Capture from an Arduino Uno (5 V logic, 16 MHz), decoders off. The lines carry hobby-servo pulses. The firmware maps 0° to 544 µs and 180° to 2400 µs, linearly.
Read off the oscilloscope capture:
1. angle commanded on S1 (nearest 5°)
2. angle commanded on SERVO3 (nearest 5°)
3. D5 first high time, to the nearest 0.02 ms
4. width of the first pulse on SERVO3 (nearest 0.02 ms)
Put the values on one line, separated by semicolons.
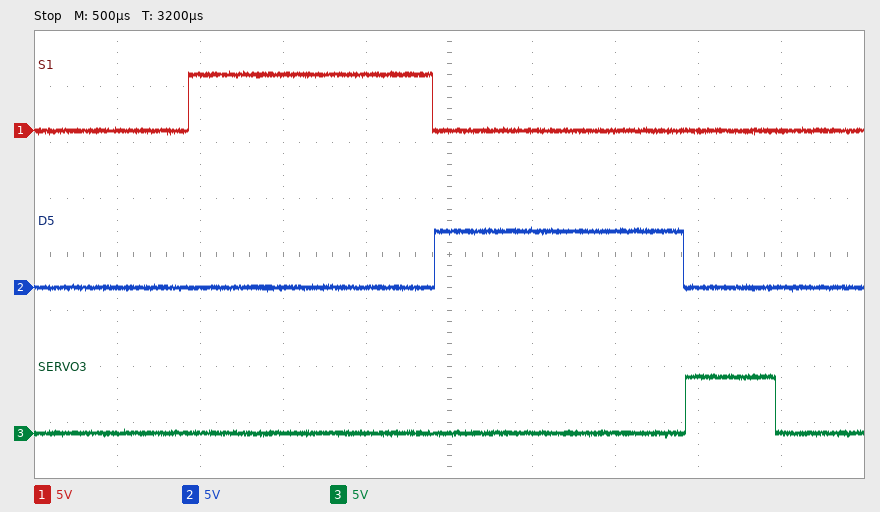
90°; 0°; 1.50 ms; 0.54 ms
